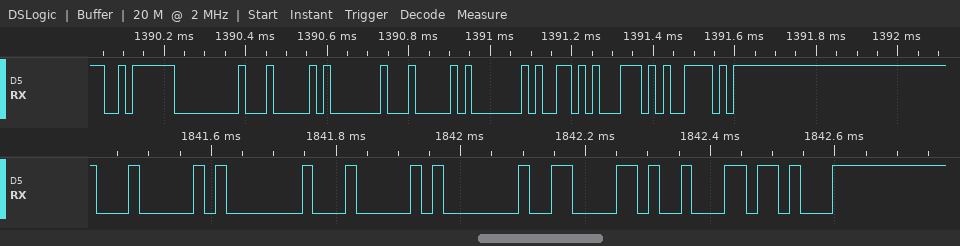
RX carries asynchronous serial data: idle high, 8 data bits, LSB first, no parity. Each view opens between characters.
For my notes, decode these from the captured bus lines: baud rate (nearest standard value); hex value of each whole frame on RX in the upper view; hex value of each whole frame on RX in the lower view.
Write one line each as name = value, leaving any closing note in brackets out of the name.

baud rate = 57600 baud
hex value of each whole frame on RX in the upper view = FA, 00, 04, 01, 04, 01, 59, 5C, 5E
hex value of each whole frame on RX in the lower view = 04, 01, 04, 01, 86, 89, 8B
